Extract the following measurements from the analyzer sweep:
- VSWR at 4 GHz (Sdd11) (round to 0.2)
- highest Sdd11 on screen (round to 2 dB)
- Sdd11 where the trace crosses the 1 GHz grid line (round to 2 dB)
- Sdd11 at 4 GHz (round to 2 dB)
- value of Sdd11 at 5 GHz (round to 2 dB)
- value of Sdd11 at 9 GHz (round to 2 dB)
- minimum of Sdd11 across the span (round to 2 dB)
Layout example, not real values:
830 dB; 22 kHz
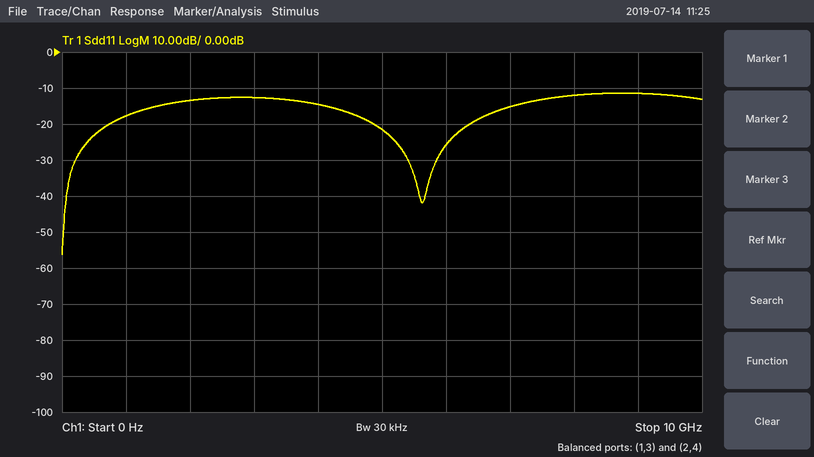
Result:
1.4; -12 dB; -18 dB; -14 dB; -22 dB; -12 dB; -56 dB
